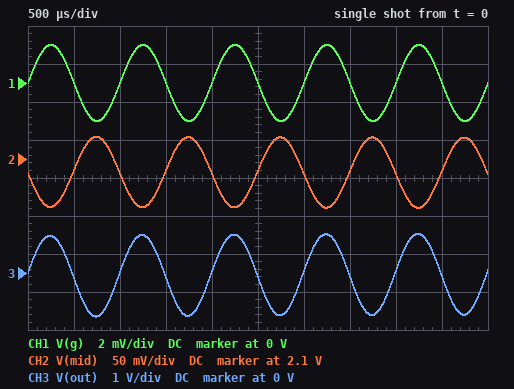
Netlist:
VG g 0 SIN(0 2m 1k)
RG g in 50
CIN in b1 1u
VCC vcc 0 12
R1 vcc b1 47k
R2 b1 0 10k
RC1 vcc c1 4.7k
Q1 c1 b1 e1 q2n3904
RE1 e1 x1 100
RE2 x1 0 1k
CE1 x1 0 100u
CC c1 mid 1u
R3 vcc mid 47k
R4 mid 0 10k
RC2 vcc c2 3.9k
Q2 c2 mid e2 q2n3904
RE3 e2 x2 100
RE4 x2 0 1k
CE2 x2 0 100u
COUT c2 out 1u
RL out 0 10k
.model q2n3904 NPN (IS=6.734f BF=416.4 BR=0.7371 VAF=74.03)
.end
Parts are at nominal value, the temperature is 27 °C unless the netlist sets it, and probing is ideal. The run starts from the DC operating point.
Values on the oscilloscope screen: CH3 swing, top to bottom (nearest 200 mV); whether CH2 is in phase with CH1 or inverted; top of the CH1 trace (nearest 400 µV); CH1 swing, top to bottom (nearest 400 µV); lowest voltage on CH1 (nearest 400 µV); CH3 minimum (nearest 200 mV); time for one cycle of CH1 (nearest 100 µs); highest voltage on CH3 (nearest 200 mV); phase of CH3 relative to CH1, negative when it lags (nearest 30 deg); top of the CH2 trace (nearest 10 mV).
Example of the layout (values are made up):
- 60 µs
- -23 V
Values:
- 2.2 V
- inverted
- 2.0 mV
- 4.0 mV
- -2.0 mV
- -1.2 V
- 1.0 ms
- 1.0 V
- 0 deg
- 2.13 V
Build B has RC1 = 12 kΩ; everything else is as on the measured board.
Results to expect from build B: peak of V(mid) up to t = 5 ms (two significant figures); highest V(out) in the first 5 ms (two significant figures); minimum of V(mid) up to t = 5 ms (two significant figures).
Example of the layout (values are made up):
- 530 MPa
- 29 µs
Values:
- 2.1 V
- 68 mV
- 2.1 V
